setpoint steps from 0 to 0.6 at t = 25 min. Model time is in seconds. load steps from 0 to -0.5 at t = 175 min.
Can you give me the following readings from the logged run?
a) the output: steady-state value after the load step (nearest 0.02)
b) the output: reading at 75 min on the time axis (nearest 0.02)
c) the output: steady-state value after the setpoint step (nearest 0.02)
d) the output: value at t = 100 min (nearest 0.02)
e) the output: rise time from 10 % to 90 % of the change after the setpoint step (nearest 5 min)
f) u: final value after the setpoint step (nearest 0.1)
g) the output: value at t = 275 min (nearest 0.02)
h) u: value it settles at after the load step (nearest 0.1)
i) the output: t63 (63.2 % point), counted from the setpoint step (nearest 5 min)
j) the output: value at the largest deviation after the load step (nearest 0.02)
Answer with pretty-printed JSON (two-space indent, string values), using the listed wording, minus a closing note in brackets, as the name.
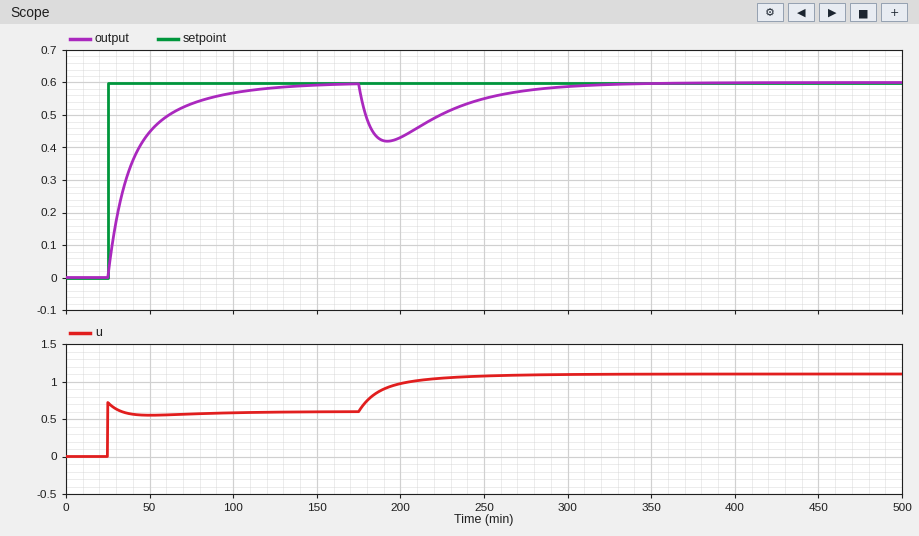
{
  "the output: steady-state value after the load step": "0.60",
  "the output: reading at 75 min on the time axis": "0.54",
  "the output: steady-state value after the setpoint step": "0.60",
  "the output: value at t = 100 min": "0.56",
  "the output: rise time from 10 % to 90 % of the change after the setpoint step": "50 min",
  "u: final value after the setpoint step": "0.6",
  "the output: value at t = 275 min": "0.58",
  "u: value it settles at after the load step": "1.1",
  "the output: t63 (63.2 % point), counted from the setpoint step": "15 min",
  "the output: value at the largest deviation after the load step": "0.42"
}
